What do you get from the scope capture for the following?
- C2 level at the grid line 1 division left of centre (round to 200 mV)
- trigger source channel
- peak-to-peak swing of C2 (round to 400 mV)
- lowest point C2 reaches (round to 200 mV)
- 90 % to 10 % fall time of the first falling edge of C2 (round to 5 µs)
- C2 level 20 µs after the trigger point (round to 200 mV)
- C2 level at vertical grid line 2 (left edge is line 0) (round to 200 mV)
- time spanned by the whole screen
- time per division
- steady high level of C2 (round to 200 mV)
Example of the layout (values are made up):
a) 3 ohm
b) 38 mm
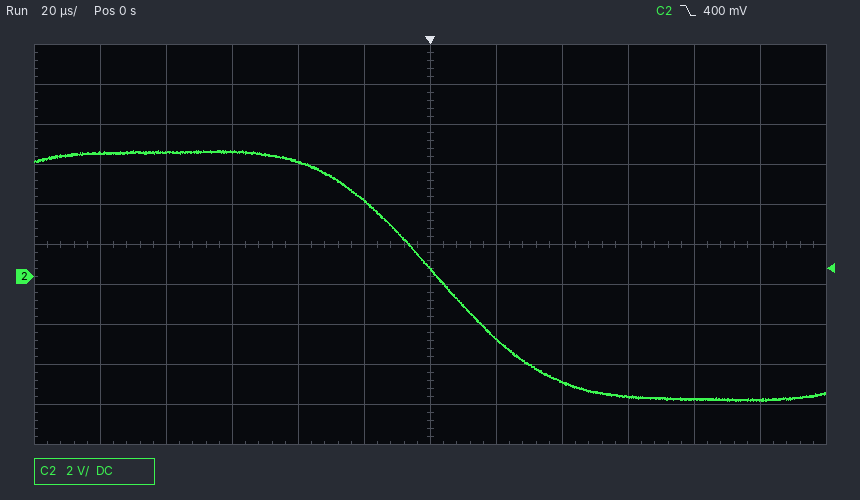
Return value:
a) 3.8 V
b) C2
c) 12.4 V
d) -6.2 V
e) 65 µs
f) -3.2 V
g) 6.2 V
h) 240 µs
i) 20 µs
j) 6.2 V
